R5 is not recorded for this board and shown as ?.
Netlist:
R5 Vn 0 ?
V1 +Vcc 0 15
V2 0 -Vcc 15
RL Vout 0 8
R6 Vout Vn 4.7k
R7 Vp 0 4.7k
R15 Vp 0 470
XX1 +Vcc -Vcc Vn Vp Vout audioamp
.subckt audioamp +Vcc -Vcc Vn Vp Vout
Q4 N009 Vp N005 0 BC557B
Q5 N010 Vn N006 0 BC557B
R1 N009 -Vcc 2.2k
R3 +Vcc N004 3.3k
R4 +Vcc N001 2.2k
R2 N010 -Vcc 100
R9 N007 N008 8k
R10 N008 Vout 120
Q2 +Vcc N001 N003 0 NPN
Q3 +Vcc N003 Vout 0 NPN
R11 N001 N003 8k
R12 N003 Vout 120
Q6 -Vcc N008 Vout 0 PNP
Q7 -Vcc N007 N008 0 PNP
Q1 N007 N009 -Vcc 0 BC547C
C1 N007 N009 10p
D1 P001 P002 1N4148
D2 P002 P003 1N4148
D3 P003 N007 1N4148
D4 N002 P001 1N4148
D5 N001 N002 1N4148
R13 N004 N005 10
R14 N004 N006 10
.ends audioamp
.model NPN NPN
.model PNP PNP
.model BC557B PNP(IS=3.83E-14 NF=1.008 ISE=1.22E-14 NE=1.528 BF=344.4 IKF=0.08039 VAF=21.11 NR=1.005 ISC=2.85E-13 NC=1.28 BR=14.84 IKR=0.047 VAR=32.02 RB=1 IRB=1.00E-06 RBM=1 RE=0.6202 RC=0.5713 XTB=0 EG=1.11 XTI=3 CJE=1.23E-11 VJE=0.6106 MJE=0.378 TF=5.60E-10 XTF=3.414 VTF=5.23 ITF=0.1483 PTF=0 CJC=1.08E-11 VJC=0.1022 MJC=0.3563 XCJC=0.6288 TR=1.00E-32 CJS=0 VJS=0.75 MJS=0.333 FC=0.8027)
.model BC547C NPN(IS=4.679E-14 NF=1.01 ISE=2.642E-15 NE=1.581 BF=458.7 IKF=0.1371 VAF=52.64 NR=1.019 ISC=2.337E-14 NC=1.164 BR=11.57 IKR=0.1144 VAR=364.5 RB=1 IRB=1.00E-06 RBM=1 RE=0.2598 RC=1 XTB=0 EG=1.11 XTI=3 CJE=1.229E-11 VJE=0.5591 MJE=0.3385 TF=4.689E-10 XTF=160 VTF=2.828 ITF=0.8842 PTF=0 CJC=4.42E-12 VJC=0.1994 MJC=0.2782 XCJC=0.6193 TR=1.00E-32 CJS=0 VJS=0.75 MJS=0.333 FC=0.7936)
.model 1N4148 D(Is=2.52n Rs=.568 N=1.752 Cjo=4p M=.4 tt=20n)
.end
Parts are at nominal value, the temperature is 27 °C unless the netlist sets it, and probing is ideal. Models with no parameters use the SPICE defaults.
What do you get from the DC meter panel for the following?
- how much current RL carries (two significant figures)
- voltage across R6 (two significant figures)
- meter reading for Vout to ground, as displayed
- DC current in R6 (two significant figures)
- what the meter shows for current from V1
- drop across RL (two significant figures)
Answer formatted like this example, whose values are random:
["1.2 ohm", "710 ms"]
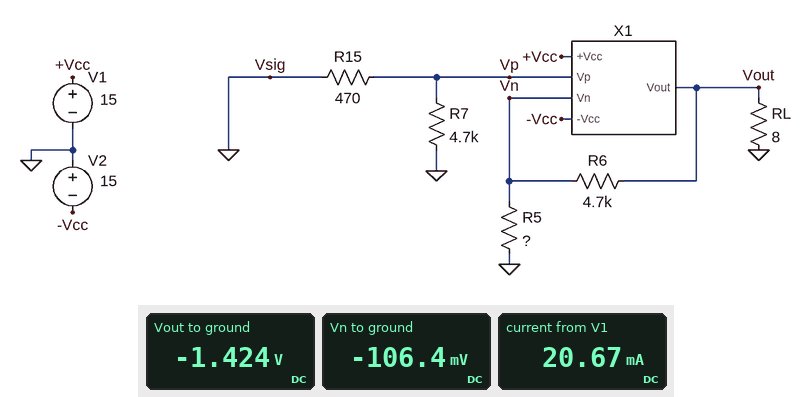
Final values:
["180 mA", "1.3 V", "-1.424 V", "280 µA", "20.67 mA", "1.4 V"]
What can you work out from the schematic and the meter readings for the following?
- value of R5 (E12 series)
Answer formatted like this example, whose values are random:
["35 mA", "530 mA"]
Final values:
["390 Ω"]
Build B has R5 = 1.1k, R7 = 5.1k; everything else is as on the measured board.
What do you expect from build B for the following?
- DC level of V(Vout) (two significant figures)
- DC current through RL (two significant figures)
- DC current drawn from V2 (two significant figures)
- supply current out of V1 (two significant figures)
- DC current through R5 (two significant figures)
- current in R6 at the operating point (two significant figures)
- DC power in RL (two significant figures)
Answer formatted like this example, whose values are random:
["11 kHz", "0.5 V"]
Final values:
["-600 mV", "75 mA", "97 mA", "22 mA", "97 µA", "100 µA", "45 mW"]
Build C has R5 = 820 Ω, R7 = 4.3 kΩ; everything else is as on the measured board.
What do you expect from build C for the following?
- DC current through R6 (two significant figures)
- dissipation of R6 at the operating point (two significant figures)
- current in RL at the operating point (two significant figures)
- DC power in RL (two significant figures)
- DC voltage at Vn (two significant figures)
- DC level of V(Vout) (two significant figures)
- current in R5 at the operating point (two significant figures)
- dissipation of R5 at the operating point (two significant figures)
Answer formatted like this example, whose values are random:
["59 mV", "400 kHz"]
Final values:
["140 µA", "89 µW", "94 mA", "71 mW", "-110 mV", "-750 mV", "130 µA", "14 µW"]
